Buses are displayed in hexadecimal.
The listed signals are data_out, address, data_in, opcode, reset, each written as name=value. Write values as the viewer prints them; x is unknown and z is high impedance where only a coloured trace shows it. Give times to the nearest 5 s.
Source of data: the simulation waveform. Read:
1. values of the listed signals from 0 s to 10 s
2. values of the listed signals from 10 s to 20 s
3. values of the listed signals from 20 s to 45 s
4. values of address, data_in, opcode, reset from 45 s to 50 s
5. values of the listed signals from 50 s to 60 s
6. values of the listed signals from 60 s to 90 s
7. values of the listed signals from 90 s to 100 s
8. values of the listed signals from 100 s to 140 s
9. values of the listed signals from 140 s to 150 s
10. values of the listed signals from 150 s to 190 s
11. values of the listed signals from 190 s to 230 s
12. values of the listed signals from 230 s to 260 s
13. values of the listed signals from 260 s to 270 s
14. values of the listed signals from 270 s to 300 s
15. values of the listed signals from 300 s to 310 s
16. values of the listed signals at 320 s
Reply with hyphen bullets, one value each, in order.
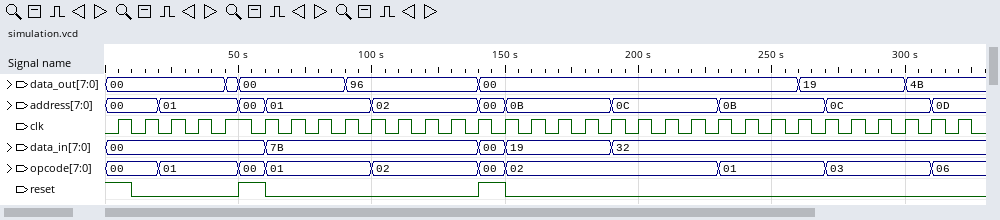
- data_out=00, address=00, data_in=00, opcode=00, reset=1
- data_out=00, address=00, data_in=00, opcode=00, reset=0
- data_out=00, address=01, data_in=00, opcode=01, reset=0
- address=01, data_in=00, opcode=01, reset=0
- data_out=00, address=00, data_in=00, opcode=00, reset=1
- data_out=00, address=01, data_in=7B, opcode=01, reset=0
- data_out=96, address=01, data_in=7B, opcode=01, reset=0
- data_out=96, address=02, data_in=7B, opcode=02, reset=0
- data_out=00, address=00, data_in=00, opcode=00, reset=1
- data_out=00, address=0B, data_in=19, opcode=02, reset=0
- data_out=00, address=0C, data_in=32, opcode=02, reset=0
- data_out=00, address=0B, data_in=32, opcode=01, reset=0
- data_out=19, address=0B, data_in=32, opcode=01, reset=0
- data_out=19, address=0C, data_in=32, opcode=03, reset=0
- data_out=4B, address=0C, data_in=32, opcode=03, reset=0
- data_out=4B, address=0D, data_in=32, opcode=06, reset=0
